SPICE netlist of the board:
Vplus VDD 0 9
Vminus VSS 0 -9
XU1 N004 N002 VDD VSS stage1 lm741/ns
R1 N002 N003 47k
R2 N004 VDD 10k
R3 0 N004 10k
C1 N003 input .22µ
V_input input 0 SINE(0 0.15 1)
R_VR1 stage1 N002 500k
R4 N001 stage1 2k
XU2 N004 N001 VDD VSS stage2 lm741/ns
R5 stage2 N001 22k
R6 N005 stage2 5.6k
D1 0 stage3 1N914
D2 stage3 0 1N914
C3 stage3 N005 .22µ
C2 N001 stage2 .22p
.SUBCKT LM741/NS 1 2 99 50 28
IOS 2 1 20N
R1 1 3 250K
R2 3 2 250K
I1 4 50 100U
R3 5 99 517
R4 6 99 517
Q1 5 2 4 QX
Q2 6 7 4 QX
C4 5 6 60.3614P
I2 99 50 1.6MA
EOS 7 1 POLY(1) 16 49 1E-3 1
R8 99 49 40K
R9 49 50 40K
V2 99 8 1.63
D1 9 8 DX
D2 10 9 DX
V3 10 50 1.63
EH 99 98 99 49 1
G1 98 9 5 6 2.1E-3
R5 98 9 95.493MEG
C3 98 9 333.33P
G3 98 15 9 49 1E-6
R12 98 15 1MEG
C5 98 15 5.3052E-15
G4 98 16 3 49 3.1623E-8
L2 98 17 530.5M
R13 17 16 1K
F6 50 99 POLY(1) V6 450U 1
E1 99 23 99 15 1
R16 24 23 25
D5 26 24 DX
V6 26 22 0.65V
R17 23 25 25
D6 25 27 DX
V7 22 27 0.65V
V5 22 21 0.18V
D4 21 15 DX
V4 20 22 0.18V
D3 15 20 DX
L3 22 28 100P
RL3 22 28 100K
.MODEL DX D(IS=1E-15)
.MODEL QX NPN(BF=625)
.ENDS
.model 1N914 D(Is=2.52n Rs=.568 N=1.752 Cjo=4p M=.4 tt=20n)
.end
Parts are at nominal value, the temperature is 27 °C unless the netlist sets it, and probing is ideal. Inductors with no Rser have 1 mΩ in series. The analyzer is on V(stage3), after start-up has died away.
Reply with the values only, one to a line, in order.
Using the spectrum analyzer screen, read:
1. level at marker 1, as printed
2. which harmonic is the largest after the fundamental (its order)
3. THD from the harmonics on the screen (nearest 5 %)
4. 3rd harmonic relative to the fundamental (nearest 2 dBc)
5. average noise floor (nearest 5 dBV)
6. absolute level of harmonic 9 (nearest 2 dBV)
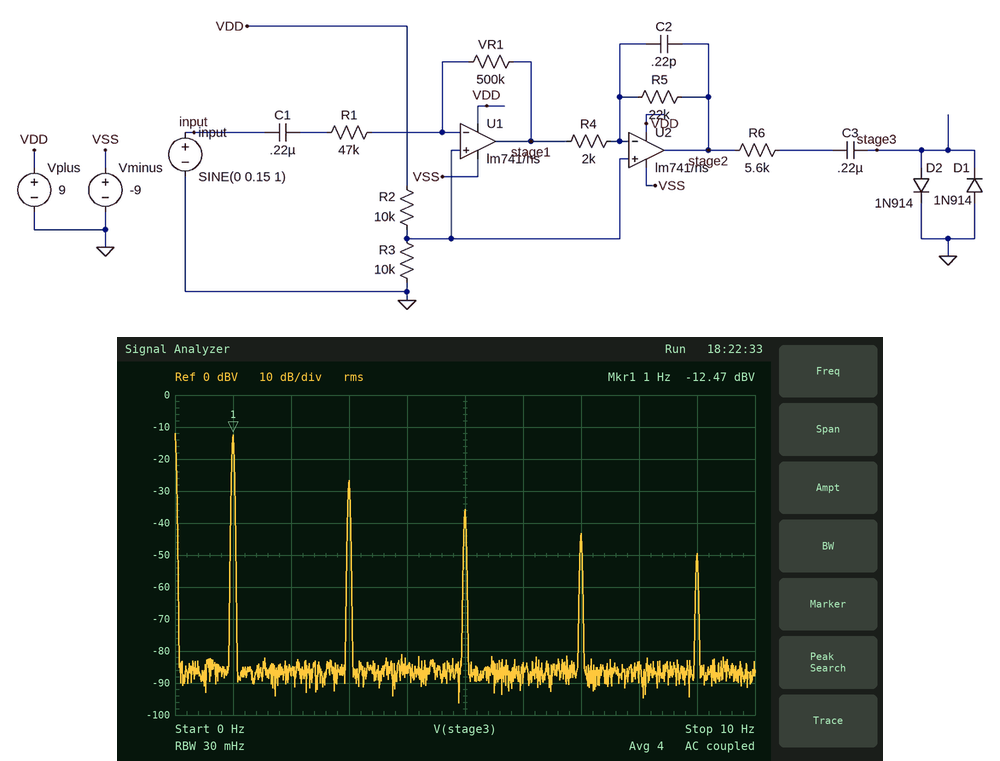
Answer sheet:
-12.47 dBV
3
20 %
-14 dBc
-85 dBV
-50 dBV
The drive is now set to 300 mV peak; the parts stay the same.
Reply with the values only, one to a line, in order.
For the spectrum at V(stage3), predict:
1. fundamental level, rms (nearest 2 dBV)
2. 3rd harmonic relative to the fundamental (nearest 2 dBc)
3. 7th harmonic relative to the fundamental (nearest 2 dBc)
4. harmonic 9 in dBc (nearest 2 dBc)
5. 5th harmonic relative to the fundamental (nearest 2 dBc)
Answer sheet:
-12 dBV
-12 dBc
-26 dBc
-32 dBc
-20 dBc
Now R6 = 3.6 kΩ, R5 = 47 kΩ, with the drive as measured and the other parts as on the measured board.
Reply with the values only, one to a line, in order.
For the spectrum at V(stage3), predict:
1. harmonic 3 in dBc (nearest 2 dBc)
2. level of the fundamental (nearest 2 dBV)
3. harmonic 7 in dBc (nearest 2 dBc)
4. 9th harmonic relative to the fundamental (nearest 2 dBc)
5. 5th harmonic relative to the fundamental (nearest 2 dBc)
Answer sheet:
-12 dBc
-12 dBV
-26 dBc
-32 dBc
-20 dBc
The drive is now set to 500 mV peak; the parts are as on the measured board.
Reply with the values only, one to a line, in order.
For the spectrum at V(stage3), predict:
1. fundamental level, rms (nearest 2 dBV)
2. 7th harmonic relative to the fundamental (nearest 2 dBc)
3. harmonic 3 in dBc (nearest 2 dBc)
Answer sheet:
-10 dBV
-24 dBc
-12 dBc
